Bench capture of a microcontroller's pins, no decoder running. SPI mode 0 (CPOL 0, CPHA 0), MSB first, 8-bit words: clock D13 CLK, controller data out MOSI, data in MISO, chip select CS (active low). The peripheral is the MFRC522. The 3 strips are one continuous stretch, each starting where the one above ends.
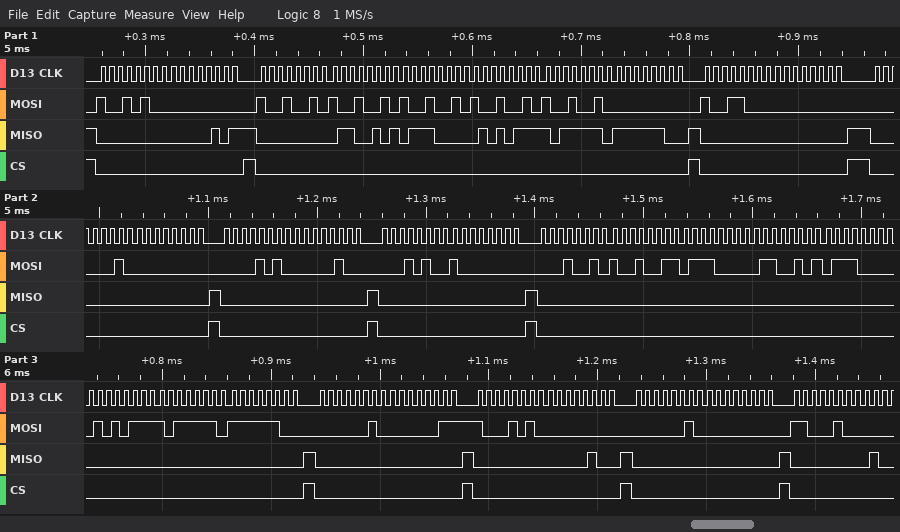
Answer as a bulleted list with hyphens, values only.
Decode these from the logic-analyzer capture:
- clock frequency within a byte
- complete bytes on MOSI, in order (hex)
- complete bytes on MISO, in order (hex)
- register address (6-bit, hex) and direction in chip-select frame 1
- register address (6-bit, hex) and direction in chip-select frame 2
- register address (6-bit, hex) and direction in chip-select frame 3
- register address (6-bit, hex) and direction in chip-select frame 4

- 125 kHz
- 94 00 92 92 92 92 92 00 98 00 02 00 0A 04 14 80 12 93 70 65 70 57 BE FC 02 03 8A 00 02 00 C4
- 00 05 00 65 70 57 BE FC 00 00 00 00 00 00 00 00 00 00 00 00 00 00 00 00 00 00 00 04 00 00 00
- 0x0A read
- 0x09 read
- 0x0C read
- 0x01 write
